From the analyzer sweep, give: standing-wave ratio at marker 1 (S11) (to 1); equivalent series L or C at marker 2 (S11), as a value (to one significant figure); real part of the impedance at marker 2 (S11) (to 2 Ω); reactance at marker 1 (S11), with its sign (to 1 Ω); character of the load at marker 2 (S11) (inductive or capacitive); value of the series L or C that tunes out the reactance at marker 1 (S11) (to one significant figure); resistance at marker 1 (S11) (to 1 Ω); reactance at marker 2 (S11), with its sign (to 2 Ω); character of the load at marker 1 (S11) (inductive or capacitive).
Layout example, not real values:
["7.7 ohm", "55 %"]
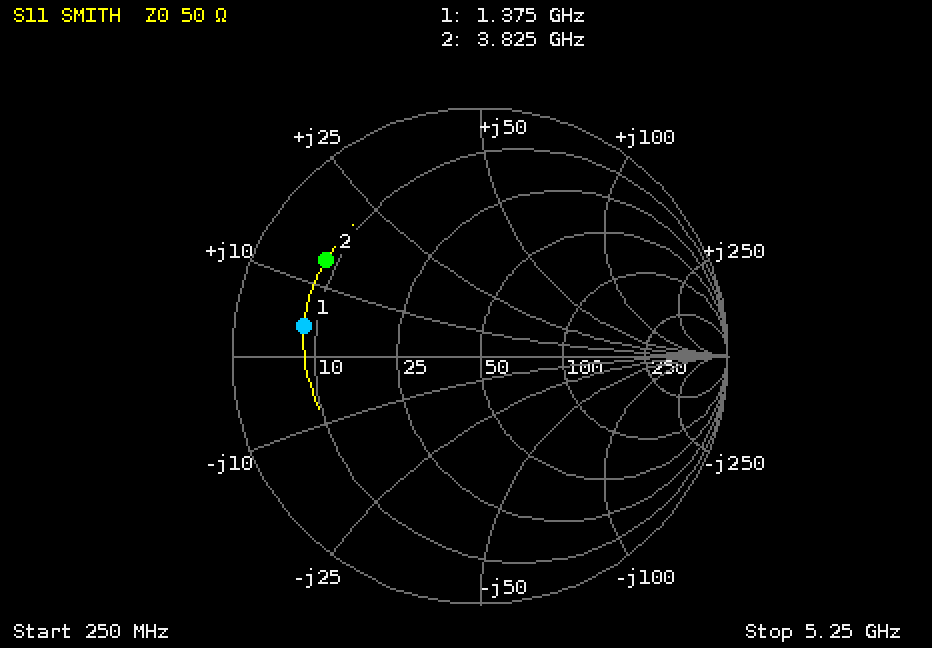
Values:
["6", "600 pH", "8 Ω", "+4 Ω", "inductive", "30 pF", "8 Ω", "+14 Ω", "inductive"]
